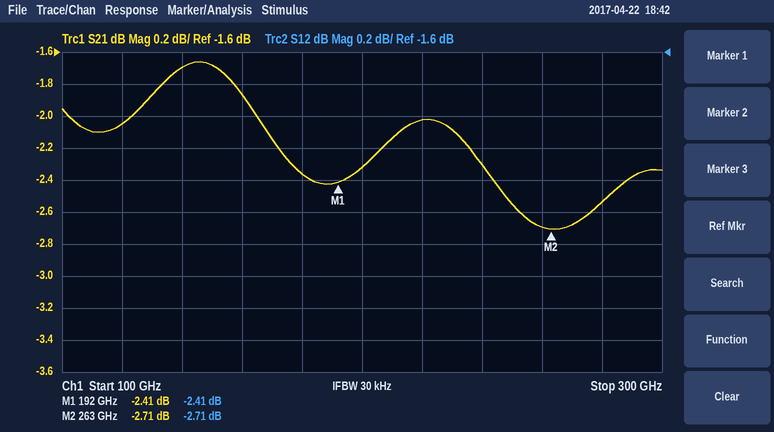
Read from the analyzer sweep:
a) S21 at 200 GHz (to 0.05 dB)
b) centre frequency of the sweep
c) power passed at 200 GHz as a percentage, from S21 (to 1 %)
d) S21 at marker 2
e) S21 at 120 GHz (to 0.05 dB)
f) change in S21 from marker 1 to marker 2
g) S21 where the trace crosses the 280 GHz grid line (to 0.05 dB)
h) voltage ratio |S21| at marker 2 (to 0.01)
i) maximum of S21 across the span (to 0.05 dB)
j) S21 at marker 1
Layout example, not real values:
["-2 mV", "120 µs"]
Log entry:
["-2.30 dB", "200 GHz", "59 %", "-2.71 dB", "-2.05 dB", "-0.30 dB", "-2.55 dB", "0.73", "-1.65 dB", "-2.41 dB"]
